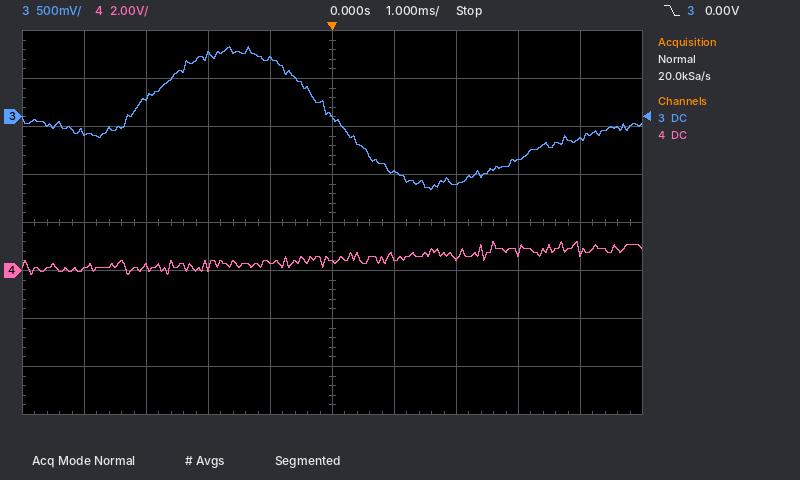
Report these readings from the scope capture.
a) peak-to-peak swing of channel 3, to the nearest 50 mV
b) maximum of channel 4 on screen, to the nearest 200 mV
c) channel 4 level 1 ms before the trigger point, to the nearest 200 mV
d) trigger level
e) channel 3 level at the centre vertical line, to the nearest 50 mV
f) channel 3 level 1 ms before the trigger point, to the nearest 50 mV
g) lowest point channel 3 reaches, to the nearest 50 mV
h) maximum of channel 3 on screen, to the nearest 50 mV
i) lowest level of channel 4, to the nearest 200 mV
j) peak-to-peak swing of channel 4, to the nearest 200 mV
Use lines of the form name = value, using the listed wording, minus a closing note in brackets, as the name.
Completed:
peak-to-peak swing of channel 3, to the nearest 50 mV = 1.50 V
maximum of channel 4 on screen, to the nearest 200 mV = 1.2 V
channel 4 level 1 ms before the trigger point, to the nearest 200 mV = 400 mV
trigger level = 0.00 V
channel 3 level at the centre vertical line, to the nearest 50 mV = 0 mV
channel 3 level 1 ms before the trigger point, to the nearest 50 mV = 600 mV
lowest point channel 3 reaches, to the nearest 50 mV = -750 mV
maximum of channel 3 on screen, to the nearest 50 mV = 750 mV
lowest level of channel 4, to the nearest 200 mV = -200 mV
peak-to-peak swing of channel 4, to the nearest 200 mV = 1.4 V
